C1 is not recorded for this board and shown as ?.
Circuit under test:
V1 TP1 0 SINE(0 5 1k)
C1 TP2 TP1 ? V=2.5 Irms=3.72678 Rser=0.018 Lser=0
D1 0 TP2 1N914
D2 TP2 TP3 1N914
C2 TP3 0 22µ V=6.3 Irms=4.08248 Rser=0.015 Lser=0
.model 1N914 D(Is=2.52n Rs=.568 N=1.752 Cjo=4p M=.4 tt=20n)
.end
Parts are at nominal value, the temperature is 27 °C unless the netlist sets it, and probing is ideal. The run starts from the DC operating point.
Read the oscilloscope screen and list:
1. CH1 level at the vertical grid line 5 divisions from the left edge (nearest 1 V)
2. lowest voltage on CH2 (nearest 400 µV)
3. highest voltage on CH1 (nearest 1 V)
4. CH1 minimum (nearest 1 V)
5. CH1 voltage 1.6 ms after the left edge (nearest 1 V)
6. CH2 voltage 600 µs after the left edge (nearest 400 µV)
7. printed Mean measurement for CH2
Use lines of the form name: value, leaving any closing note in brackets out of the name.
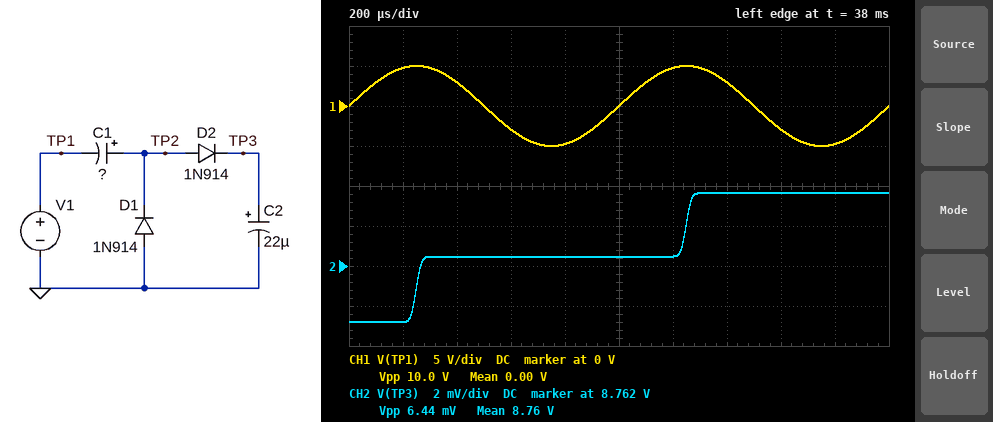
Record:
CH1 level at the vertical grid line 5 divisions from the left edge: 0 V
lowest voltage on CH2: 8.7592 V
highest voltage on CH1: 5 V
CH1 minimum: -5 V
CH1 voltage 1.6 ms after the left edge: -3 V
CH2 voltage 600 µs after the left edge: 8.7624 V
printed Mean measurement for CH2: 8.76 V
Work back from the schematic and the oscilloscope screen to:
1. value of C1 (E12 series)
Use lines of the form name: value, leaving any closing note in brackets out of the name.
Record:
value of C1: 12 µF
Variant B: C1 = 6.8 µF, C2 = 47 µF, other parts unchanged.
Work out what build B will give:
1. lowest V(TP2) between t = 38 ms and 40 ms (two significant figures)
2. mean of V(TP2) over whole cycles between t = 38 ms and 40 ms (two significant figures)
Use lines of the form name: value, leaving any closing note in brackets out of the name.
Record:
lowest V(TP2) between t = 38 ms and 40 ms: -700 mV
mean of V(TP2) over whole cycles between t = 38 ms and 40 ms: 4.3 V
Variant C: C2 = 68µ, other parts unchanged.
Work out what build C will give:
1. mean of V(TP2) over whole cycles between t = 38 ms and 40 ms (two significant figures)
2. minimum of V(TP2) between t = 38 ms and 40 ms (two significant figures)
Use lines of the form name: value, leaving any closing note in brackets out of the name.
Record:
mean of V(TP2) over whole cycles between t = 38 ms and 40 ms: 4.3 V
minimum of V(TP2) between t = 38 ms and 40 ms: -710 mV
